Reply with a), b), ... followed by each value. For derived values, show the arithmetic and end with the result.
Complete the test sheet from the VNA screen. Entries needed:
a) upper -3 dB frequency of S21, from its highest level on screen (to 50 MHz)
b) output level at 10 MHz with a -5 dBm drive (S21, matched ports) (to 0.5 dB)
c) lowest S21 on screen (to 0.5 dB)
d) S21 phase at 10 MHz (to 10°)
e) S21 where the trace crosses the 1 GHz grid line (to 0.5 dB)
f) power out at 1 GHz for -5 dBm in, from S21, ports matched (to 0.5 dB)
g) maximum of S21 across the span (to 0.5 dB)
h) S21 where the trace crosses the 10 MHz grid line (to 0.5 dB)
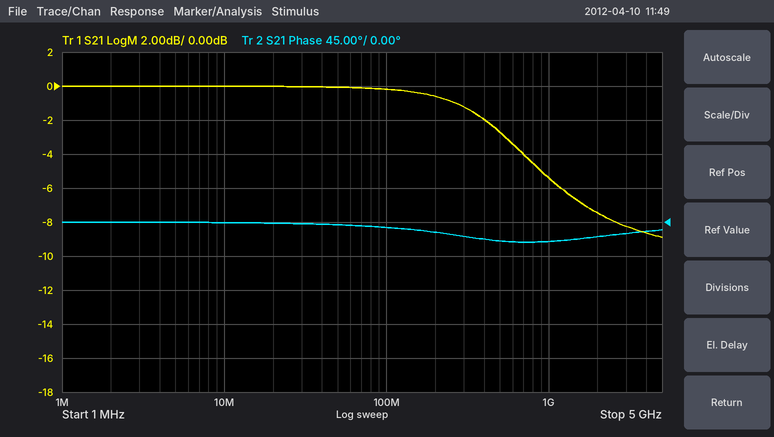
a) 550 MHz
b) -5 dBm + (0.0 dB) = -5.0 dBm
c) -9.0 dB
d) 0°
e) -5.5 dB
f) -5 dBm + (-5.5 dB) = -10.5 dBm
g) 0.0 dB
h) 0.0 dB
